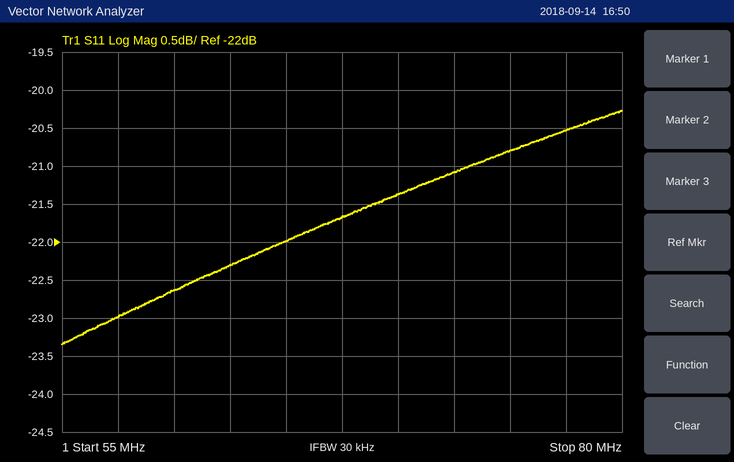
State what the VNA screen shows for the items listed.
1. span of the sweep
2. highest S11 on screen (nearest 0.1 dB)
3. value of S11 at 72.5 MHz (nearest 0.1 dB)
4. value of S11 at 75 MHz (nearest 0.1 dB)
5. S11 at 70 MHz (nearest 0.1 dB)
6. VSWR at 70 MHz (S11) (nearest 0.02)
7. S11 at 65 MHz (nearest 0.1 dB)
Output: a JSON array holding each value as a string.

["25 MHz", "-20.3 dB", "-21.1 dB", "-20.8 dB", "-21.4 dB", "1.18", "-22.0 dB"]
